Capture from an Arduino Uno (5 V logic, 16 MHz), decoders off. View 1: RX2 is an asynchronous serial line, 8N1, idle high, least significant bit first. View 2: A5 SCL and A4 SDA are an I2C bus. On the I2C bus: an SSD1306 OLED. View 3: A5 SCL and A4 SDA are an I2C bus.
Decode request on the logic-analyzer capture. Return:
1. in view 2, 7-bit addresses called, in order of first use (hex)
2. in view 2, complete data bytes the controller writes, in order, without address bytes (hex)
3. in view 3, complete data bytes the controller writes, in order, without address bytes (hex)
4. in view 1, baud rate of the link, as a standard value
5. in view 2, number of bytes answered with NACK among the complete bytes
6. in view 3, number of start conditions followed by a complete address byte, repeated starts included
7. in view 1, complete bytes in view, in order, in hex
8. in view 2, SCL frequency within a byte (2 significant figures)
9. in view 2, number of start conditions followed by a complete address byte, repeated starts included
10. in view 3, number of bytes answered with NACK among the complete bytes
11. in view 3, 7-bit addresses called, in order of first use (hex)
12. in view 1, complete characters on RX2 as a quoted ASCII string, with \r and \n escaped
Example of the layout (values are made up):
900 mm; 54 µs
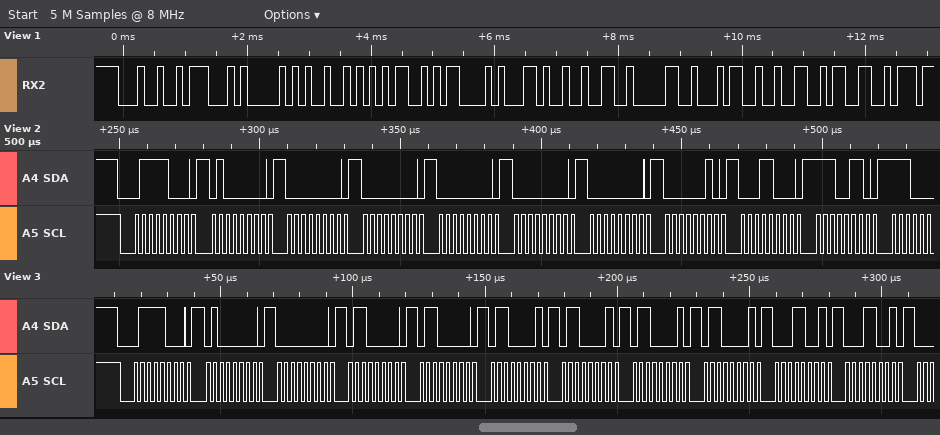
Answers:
0x3C; 40 00 00 00 00 00 02 18 E6; 40 00 60 60 61 61 61 61 19 19; 9600 baud; 0; 1; 24 47 50 52 4D 43 2C 32 30 34 32 33; 400 kHz; 1; 0; 0x3C; "$GPRMC,20423"
